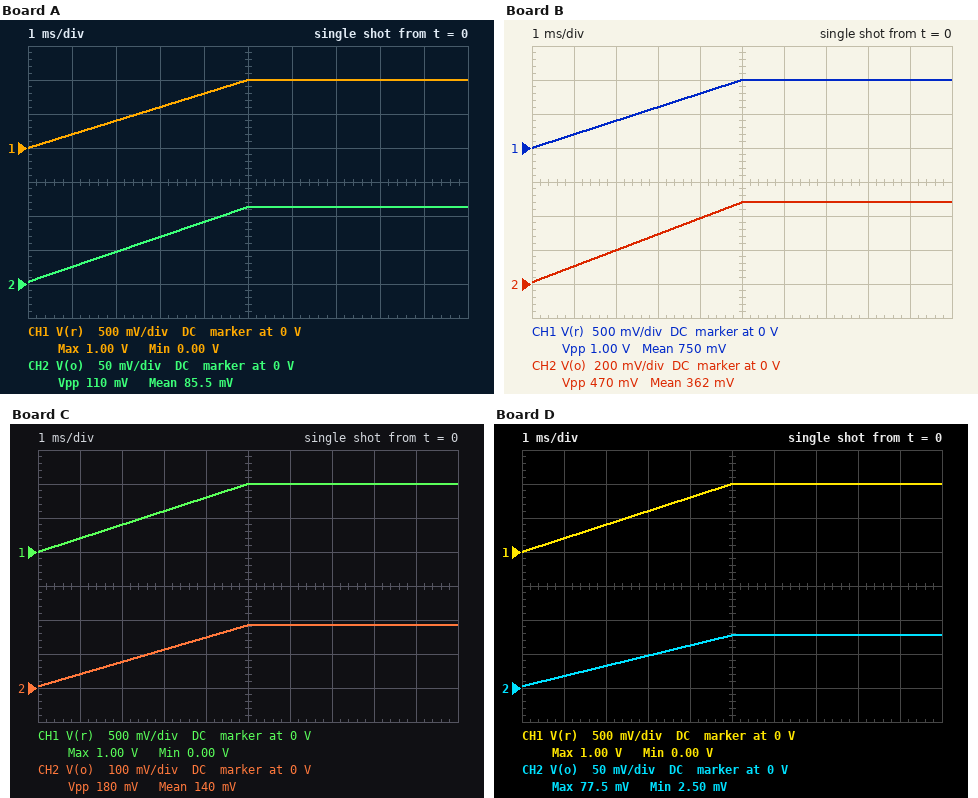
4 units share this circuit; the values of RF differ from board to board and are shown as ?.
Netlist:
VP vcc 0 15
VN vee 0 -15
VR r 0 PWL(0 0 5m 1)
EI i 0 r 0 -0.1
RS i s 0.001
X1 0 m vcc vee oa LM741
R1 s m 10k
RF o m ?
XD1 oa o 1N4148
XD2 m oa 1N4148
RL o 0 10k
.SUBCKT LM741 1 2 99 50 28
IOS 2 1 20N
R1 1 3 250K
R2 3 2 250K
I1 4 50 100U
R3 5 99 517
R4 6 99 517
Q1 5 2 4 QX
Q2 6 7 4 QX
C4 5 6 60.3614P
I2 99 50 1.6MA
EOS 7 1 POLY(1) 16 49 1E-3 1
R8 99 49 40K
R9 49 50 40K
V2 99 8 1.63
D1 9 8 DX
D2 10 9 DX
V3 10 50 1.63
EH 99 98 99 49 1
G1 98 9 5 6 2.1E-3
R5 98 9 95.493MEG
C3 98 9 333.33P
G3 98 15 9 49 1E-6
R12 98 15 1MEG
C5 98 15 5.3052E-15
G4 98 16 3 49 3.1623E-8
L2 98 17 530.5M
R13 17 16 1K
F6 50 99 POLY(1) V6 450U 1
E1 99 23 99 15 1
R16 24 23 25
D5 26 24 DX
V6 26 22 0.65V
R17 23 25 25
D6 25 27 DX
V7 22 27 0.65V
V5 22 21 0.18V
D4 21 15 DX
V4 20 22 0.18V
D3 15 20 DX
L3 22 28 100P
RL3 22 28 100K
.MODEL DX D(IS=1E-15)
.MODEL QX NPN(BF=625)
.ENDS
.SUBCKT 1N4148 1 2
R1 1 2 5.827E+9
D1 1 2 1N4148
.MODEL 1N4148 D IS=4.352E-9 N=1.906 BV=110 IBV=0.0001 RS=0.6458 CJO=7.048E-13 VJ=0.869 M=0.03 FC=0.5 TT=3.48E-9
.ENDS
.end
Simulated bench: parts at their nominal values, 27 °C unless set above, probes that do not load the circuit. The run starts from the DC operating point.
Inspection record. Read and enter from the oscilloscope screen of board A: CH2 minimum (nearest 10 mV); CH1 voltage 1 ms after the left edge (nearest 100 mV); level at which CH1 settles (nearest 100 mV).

0 V
200 mV
1.0 V
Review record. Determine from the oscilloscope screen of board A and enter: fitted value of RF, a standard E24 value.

11 kΩ
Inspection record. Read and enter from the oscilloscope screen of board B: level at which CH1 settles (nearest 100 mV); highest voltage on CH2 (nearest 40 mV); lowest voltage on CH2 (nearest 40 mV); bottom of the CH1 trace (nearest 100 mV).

1.0 V
480 mV
0 V
0 V
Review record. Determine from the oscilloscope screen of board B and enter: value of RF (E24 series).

47 kΩ
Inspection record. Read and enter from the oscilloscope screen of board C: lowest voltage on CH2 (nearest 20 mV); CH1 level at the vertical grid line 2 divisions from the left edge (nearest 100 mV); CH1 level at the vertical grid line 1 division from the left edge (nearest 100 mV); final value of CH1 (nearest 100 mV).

0 V
400 mV
200 mV
1.0 V
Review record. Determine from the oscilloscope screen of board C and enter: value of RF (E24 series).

18 kΩ
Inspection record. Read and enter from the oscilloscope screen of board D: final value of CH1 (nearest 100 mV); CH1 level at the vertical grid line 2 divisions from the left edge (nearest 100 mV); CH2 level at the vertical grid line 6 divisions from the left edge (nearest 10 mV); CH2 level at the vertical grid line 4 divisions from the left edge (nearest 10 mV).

1.0 V
400 mV
80 mV
60 mV
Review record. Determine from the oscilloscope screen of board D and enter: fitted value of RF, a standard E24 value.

7.5 kΩ
